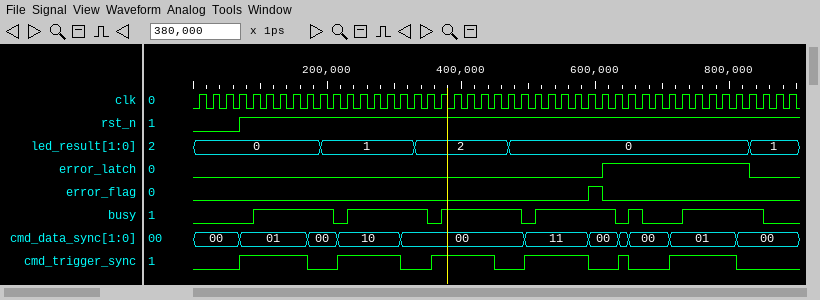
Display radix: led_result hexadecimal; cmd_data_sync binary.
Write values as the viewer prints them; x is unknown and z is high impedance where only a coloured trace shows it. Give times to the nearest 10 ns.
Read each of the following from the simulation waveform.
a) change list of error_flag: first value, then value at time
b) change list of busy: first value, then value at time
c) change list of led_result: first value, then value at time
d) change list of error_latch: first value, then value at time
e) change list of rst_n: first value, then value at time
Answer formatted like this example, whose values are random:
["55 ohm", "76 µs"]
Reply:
["0, 1 at 590 ns, 0 at 610 ns", "0, 1 at 90 ns, 0 at 210 ns, 1 at 230 ns, 0 at 350 ns, 1 at 370 ns, 0 at 490 ns, 1 at 510 ns, 0 at 630 ns, 1 at 650 ns, 0 at 670 ns, 1 at 730 ns, 0 at 850 ns", "0, 1 at 190 ns, 2 at 330 ns, 0 at 470 ns, 1 at 830 ns", "0, 1 at 610 ns, 0 at 830 ns", "0, 1 at 70 ns"]
